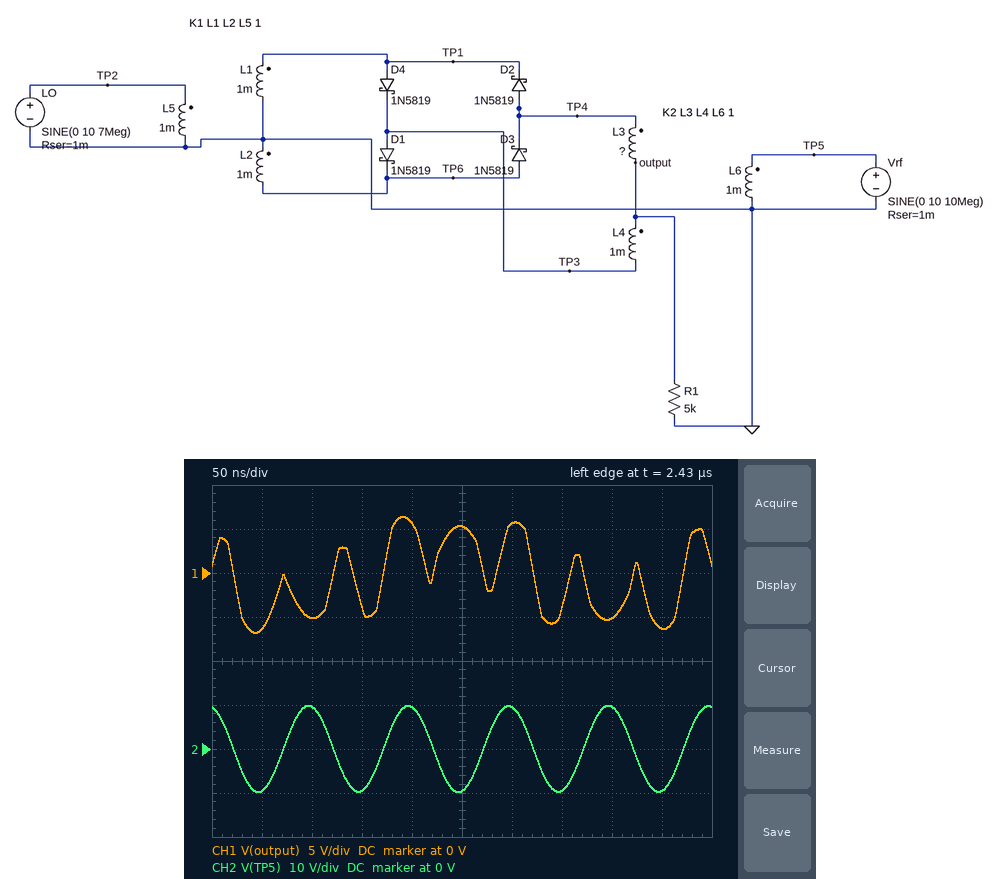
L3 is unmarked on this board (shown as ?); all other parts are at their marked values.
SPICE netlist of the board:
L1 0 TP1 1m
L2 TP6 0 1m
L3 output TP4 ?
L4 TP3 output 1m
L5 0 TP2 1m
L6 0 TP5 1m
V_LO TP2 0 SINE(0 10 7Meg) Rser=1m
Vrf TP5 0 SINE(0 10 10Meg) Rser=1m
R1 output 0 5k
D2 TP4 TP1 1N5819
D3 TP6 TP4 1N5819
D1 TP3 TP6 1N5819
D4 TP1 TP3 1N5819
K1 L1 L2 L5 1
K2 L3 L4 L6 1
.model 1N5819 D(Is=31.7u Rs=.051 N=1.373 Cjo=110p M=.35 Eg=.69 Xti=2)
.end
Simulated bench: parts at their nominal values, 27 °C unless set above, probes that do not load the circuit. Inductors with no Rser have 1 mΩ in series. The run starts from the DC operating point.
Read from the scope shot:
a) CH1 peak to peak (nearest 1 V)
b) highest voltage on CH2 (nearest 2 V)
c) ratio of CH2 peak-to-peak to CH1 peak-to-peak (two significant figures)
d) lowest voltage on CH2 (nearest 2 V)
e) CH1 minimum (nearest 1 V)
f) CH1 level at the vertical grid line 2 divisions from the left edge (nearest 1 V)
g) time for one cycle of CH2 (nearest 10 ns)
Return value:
13 V
10 V
1.5
-10 V
-7 V
-5 V
100 ns
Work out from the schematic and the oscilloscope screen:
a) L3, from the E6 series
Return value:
680 µH
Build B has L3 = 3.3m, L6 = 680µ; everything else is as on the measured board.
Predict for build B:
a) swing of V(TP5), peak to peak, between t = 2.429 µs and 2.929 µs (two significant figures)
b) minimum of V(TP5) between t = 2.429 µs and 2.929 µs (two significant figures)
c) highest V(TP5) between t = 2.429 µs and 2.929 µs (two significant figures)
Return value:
18 V
-9.2 V
9.2 V
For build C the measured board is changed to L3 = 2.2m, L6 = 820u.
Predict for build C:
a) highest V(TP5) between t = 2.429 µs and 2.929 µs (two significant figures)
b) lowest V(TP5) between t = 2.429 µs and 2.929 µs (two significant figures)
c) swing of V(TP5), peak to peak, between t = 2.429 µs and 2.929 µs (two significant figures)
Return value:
9.5 V
-9.5 V
19 V
